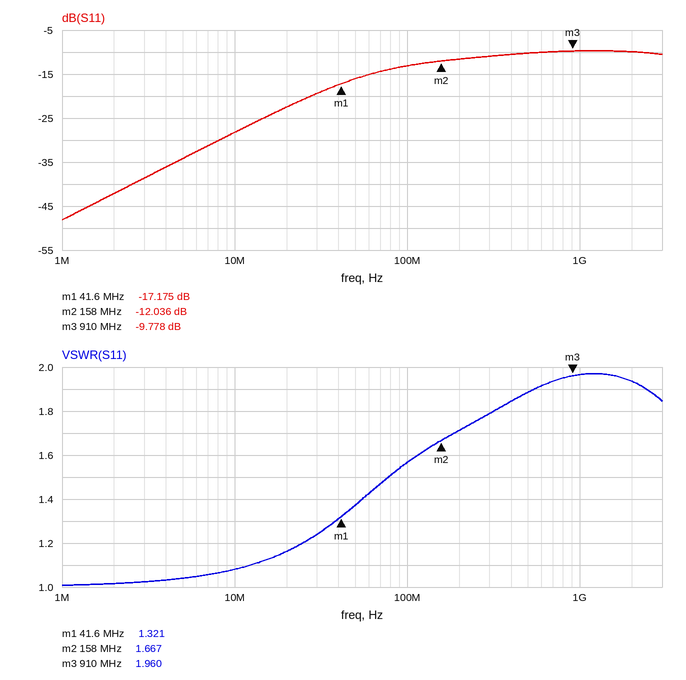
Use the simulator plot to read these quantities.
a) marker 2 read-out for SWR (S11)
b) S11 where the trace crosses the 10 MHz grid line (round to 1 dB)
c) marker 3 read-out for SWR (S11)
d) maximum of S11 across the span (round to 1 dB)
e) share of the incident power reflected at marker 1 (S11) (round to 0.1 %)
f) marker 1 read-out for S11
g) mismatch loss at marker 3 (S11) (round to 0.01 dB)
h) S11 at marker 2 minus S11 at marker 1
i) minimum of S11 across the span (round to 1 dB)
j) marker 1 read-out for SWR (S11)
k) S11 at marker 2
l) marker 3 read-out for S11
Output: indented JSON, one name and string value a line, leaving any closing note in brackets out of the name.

{
  "marker 2 read-out for SWR": "1.667",
  "S11 where the trace crosses the 10 MHz grid line": "-28 dB",
  "marker 3 read-out for SWR": "1.960",
  "maximum of S11 across the span": "-10 dB",
  "share of the incident power reflected at marker 1 (S11)": "1.9 %",
  "marker 1 read-out for S11": "-17.175 dB",
  "mismatch loss at marker 3 (S11)": "0.48 dB",
  "S11 at marker 2 minus S11 at marker 1": "5.139 dB",
  "minimum of S11 across the span": "-48 dB",
  "marker 1 read-out for SWR": "1.321",
  "S11 at marker 2": "-12.036 dB",
  "marker 3 read-out for S11": "-9.778 dB"
}
